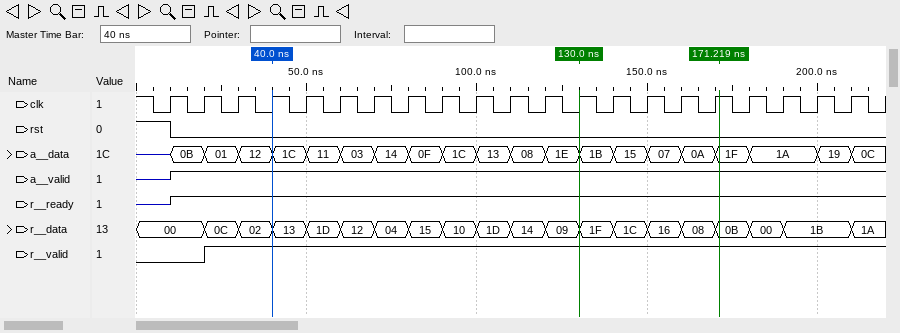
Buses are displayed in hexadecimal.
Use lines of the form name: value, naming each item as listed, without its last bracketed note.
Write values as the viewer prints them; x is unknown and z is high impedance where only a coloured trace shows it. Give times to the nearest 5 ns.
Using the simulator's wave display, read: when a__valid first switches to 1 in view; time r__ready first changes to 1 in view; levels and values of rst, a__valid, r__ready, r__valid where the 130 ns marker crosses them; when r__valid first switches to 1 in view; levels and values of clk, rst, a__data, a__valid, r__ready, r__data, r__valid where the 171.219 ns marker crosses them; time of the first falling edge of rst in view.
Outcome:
when a__valid first switches to 1 in view: 10 ns
time r__ready first changes to 1 in view: 10 ns
levels and values of rst, a__valid, r__ready, r__valid where the 130 ns marker crosses them: rst=0, a__valid=1, r__ready=1, r__valid=1
when r__valid first switches to 1 in view: 20 ns
levels and values of clk, rst, a__data, a__valid, r__ready, r__data, r__valid where the 171.219 ns marker crosses them: clk=1, rst=0, a__data=1F, a__valid=1, r__ready=1, r__data=0B, r__valid=1
time of the first falling edge of rst in view: 10 ns
